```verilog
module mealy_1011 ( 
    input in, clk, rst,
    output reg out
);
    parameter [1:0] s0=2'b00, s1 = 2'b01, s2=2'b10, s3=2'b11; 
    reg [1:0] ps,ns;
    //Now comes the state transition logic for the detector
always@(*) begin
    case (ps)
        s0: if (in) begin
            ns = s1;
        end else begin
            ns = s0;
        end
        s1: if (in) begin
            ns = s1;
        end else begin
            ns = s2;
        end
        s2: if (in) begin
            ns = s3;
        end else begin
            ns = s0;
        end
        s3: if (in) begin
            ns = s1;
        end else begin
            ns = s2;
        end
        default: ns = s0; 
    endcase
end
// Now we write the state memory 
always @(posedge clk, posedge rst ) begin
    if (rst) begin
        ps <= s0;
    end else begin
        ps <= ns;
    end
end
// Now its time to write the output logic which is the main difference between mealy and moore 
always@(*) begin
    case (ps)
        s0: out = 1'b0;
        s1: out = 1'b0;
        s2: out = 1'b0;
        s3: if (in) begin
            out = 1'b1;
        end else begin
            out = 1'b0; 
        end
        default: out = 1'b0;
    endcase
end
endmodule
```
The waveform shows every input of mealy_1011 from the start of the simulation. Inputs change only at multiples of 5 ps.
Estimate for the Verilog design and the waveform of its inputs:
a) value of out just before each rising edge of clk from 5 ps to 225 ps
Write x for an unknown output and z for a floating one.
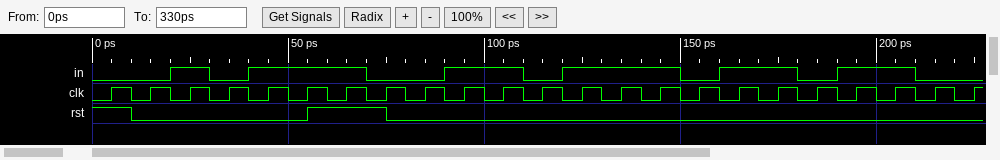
0 0 0 0 0 1 0 0 0 0 0 0 0 1 0 0 0 1 0 0 1 0 0
